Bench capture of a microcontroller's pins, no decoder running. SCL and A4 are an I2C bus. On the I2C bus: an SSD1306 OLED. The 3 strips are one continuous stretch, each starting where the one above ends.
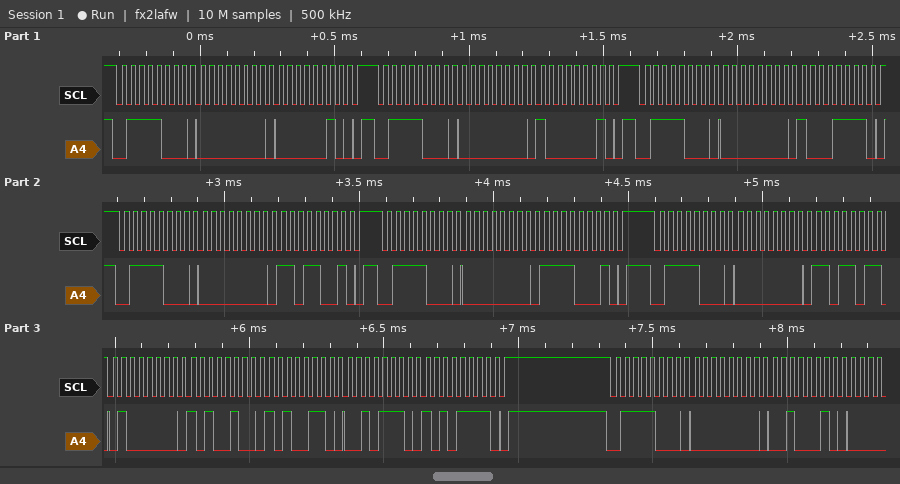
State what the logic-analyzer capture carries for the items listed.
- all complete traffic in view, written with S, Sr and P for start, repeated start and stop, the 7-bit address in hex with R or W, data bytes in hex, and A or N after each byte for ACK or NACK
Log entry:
S 3CW A 00 A 02 A P S 3CW A 00 A 81 A P S 3CW A 00 A 8F A P S 3CW A 00 A D9 A P S 3CW A 00 A F1 A P S 3CW A 00 A DB A 40 A A4 A A6 A 2E A AF A P S 3CW A 00 A 22 A
